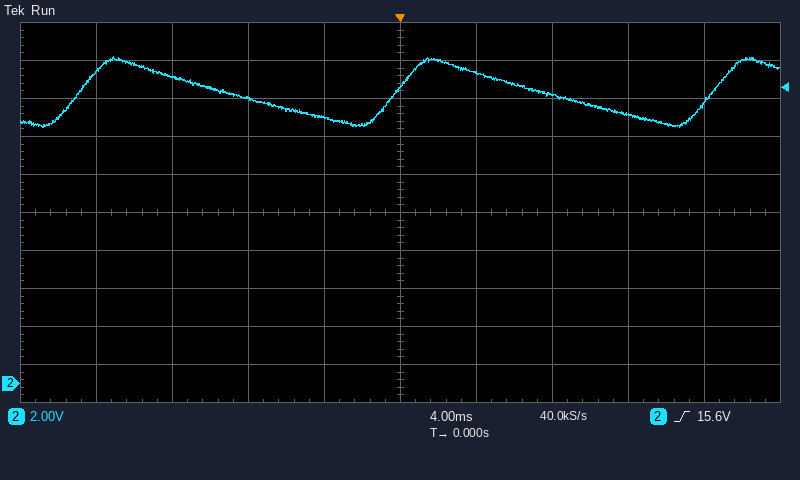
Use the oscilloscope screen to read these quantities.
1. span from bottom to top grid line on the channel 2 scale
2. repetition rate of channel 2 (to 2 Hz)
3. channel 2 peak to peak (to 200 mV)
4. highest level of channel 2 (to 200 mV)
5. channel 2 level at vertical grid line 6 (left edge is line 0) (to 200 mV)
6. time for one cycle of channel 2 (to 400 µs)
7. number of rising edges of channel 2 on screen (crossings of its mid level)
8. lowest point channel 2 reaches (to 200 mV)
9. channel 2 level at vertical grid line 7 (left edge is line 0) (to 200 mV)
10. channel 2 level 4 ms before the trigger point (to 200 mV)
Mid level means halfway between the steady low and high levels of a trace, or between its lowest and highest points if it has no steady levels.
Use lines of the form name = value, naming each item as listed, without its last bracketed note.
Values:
span from bottom to top grid line on the channel 2 scale = 20 V
repetition rate of channel 2 = 60 Hz
channel 2 peak to peak = 3.8 V
highest level of channel 2 = 17.2 V
channel 2 level at vertical grid line 6 (left edge is line 0) = 16.4 V
time for one cycle of channel 2 = 16.8 ms
number of rising edges of channel 2 on screen = 3
lowest point channel 2 reaches = 13.4 V
channel 2 level at vertical grid line 7 (left edge is line 0) = 15.2 V
channel 2 level 4 ms before the trigger point = 14.0 V
